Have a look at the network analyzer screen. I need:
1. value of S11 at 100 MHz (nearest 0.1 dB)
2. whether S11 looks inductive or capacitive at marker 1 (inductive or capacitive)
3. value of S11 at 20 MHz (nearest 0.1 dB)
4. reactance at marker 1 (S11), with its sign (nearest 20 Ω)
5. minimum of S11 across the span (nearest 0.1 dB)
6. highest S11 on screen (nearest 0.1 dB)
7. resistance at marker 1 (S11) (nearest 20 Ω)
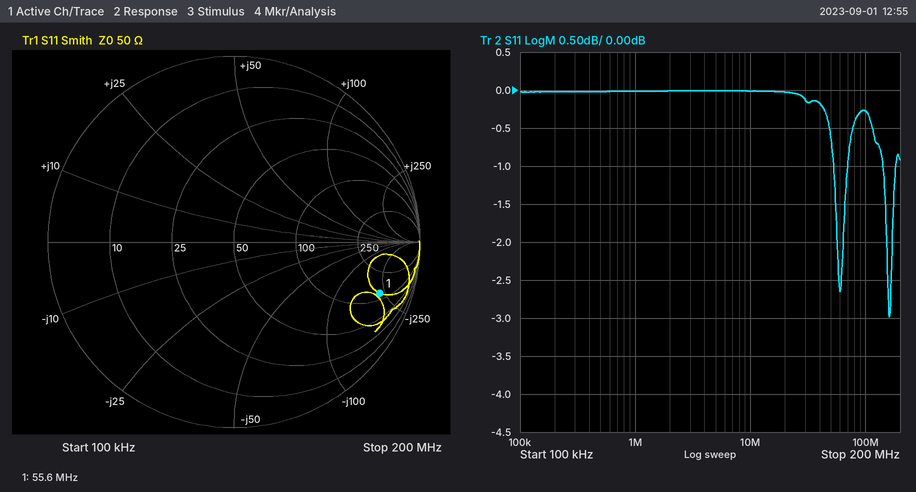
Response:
-0.3 dB
capacitive
0.0 dB
-220 Ω
-3.0 dB
0.0 dB
120 Ω
